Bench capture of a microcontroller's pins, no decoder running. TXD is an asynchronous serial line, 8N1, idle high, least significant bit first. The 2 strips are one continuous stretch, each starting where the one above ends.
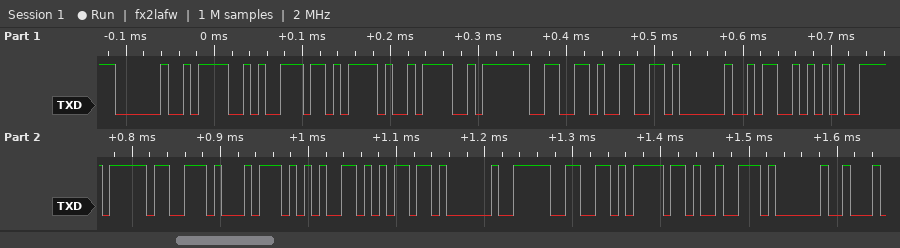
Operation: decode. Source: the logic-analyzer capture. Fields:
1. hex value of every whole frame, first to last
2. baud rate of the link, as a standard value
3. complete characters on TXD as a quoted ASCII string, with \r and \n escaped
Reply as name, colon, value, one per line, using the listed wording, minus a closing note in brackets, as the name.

hex value of every whole frame, first to last: 20 4F 6E 2F 4F 66 66 20 53 79 73 74 65 6D 20 66 6F 72 20
baud rate of the link, as a standard value: 115200 baud
complete characters on TXD as a quoted ASCII string, with \r and \n escaped: " On/Off System for "
